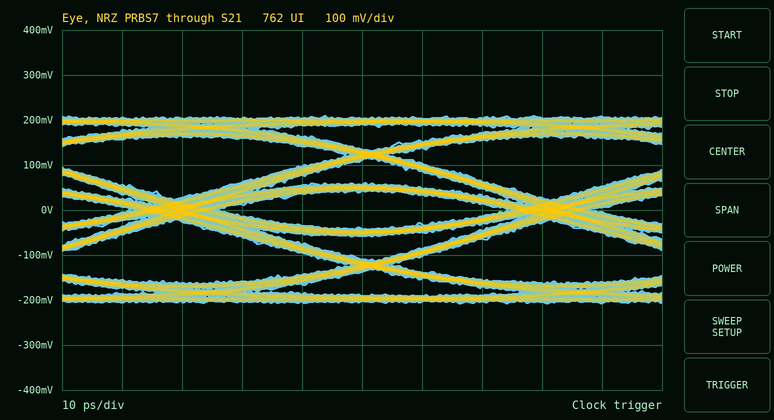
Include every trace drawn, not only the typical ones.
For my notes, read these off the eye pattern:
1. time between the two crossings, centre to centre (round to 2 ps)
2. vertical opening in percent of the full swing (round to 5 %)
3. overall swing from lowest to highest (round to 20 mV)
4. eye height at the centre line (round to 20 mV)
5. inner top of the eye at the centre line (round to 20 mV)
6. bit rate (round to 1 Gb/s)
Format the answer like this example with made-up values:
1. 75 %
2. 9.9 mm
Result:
1. 62 ps
2. 20 %
3. 420 mV
4. 80 mV
5. 40 mV
6. 16 Gb/s
